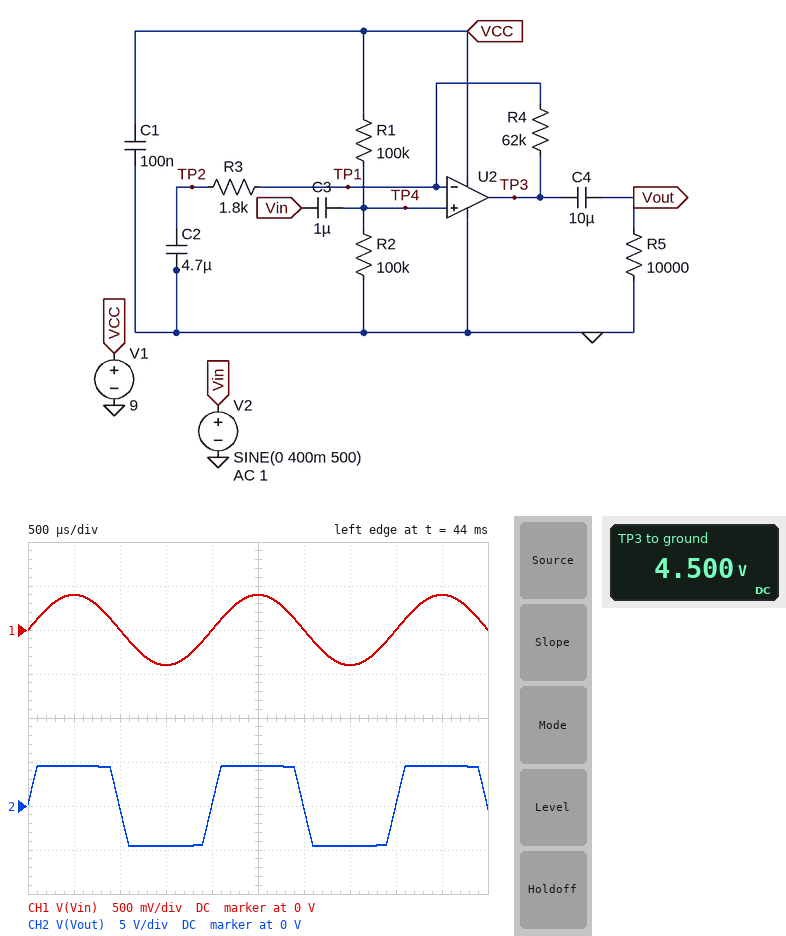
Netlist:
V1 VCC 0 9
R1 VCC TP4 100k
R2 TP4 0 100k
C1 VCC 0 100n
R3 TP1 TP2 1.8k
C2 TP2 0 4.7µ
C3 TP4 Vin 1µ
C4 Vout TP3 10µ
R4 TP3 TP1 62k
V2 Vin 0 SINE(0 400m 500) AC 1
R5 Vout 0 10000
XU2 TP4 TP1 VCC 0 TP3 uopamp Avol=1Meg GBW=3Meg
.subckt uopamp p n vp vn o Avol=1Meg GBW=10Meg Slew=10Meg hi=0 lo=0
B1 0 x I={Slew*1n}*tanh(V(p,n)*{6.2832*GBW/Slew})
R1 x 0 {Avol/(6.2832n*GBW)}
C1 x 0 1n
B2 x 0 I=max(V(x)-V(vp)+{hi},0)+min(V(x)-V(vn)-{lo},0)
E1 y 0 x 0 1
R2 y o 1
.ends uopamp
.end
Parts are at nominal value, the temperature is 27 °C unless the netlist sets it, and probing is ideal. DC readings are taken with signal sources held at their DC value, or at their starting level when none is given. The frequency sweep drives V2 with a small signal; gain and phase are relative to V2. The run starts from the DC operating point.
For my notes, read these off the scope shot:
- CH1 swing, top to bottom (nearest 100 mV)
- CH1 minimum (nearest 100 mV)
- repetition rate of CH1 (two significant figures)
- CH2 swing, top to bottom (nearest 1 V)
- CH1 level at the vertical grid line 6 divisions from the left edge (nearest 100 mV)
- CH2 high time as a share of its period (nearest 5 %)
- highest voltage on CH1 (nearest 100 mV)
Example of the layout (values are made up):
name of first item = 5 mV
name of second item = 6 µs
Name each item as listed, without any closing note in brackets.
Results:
CH1 swing, top to bottom = 800 mV
CH1 minimum = -400 mV
repetition rate of CH1 = 500 Hz
CH2 swing, top to bottom = 9 V
CH1 level at the vertical grid line 6 divisions from the left edge = 0 V
CH2 high time as a share of its period = 50 %
highest voltage on CH1 = 400 mV
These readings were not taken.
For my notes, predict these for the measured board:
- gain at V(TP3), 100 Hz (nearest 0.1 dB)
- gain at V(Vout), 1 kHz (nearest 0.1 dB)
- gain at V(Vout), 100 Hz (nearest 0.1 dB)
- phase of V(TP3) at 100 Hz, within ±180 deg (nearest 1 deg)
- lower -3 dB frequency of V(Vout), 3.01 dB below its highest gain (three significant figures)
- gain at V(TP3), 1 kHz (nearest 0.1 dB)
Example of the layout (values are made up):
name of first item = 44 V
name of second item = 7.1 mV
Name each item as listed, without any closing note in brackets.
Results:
gain at V(TP3), 100 Hz = 30.8 dB
gain at V(Vout), 1 kHz = 31.0 dB
gain at V(Vout), 100 Hz = 30.8 dB
phase of V(TP3) at 100 Hz, within ±180 deg = 12 deg
lower -3 dB frequency of V(Vout), 3.01 dB below its highest gain = 19.4 Hz
gain at V(TP3), 1 kHz = 31.0 dB
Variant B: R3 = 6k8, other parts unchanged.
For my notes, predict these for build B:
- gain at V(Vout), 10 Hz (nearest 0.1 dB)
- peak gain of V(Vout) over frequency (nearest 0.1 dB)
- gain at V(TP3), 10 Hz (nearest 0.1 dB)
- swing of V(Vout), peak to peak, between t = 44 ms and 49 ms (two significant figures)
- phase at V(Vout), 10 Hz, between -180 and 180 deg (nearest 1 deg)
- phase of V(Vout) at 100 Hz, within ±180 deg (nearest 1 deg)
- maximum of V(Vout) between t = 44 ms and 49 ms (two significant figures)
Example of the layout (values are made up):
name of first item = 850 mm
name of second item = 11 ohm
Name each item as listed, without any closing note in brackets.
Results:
gain at V(Vout), 10 Hz = 18.6 dB
peak gain of V(Vout) over frequency = 20.1 dB
gain at V(TP3), 10 Hz = 18.7 dB
swing of V(Vout), peak to peak, between t = 44 ms and 49 ms = 8.1 V
phase at V(Vout), 10 Hz, between -180 and 180 deg = 50 deg
phase of V(Vout) at 100 Hz, within ±180 deg = 5 deg
maximum of V(Vout) between t = 44 ms and 49 ms = 4.0 V
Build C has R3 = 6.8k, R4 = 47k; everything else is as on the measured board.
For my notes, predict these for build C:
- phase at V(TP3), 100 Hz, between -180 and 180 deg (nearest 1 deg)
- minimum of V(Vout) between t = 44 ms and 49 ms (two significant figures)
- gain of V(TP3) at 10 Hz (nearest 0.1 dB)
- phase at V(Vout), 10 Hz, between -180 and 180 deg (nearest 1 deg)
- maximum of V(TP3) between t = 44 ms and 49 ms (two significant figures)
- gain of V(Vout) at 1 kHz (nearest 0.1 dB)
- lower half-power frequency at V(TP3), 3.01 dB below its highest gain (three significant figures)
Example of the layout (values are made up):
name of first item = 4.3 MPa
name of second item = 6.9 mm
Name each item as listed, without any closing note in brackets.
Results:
phase at V(TP3), 100 Hz, between -180 and 180 deg = 4 deg
minimum of V(Vout) between t = 44 ms and 49 ms = -3.2 V
gain of V(TP3) at 10 Hz = 16.6 dB
phase at V(Vout), 10 Hz, between -180 and 180 deg = 50 deg
maximum of V(TP3) between t = 44 ms and 49 ms = 7.7 V
gain of V(Vout) at 1 kHz = 18.0 dB
lower half-power frequency at V(TP3), 3.01 dB below its highest gain = 6.35 Hz
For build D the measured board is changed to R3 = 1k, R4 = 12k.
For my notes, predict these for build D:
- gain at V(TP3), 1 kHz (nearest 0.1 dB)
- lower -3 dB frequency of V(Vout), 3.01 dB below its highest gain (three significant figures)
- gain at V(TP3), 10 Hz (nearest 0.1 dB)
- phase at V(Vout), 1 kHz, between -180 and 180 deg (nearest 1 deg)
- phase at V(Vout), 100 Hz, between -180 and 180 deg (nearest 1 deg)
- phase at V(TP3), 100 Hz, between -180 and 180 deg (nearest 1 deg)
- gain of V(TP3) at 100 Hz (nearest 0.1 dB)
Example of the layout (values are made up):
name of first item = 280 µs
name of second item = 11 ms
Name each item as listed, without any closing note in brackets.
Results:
gain at V(TP3), 1 kHz = 22.3 dB
lower -3 dB frequency of V(Vout), 3.01 dB below its highest gain = 34.0 Hz
gain at V(TP3), 10 Hz = 11.2 dB
phase at V(Vout), 1 kHz, between -180 and 180 deg = 2 deg
phase at V(Vout), 100 Hz, between -180 and 180 deg = 20 deg
phase at V(TP3), 100 Hz, between -180 and 180 deg = 19 deg
gain of V(TP3) at 100 Hz = 21.8 dB
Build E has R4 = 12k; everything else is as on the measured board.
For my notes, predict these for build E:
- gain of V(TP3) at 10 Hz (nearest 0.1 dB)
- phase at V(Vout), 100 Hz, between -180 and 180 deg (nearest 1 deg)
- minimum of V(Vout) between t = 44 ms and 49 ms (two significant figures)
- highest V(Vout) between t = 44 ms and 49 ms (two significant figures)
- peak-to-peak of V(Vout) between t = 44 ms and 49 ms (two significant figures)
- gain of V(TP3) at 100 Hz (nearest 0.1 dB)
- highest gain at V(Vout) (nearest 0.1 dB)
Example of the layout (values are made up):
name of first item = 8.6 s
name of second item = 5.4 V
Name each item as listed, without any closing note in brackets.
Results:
gain of V(TP3) at 10 Hz = 11.0 dB
phase at V(Vout), 100 Hz, between -180 and 180 deg = 12 deg
minimum of V(Vout) between t = 44 ms and 49 ms = -3.1 V
highest V(Vout) between t = 44 ms and 49 ms = 3.1 V
peak-to-peak of V(Vout) between t = 44 ms and 49 ms = 6.1 V
gain of V(TP3) at 100 Hz = 17.5 dB
highest gain at V(Vout) = 17.7 dB
